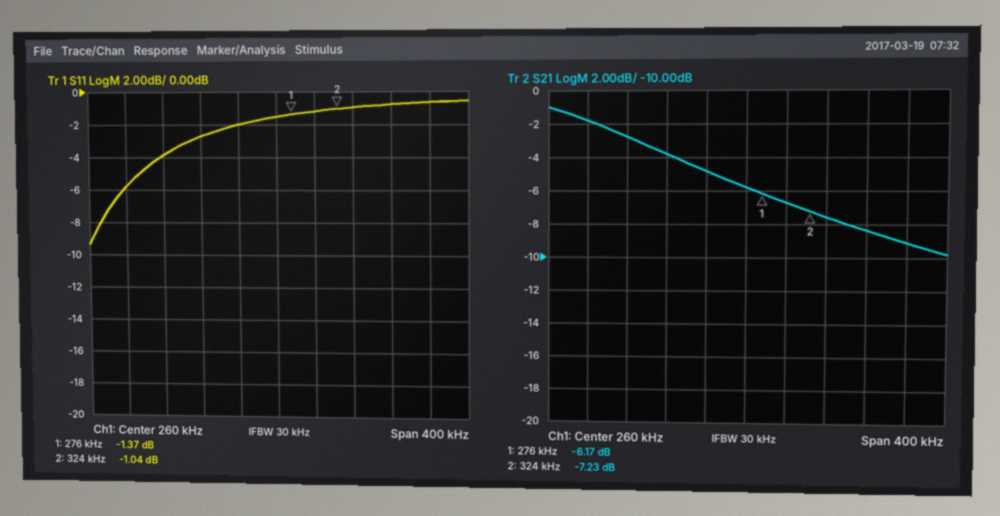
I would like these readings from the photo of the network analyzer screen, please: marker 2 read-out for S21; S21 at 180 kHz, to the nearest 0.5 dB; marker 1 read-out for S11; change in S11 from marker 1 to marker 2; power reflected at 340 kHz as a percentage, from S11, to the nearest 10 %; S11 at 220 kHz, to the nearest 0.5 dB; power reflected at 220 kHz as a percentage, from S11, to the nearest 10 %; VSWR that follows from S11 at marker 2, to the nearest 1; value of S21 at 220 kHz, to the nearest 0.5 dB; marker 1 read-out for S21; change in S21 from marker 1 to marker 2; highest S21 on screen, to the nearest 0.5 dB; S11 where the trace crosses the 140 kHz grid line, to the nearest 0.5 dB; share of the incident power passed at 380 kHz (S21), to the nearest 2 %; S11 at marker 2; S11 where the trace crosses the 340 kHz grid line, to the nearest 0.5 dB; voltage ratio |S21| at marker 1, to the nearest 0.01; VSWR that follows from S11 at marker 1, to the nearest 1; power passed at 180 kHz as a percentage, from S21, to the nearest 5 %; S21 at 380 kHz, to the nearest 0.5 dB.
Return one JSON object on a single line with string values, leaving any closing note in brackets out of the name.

{"marker 2 read-out for S21": "-7.23 dB", "S21 at 180 kHz, to the nearest 0.5 dB": "-4.0 dB", "marker 1 read-out for S11": "-1.37 dB", "change in S11 from marker 1 to marker 2": "0.33 dB", "power reflected at 340 kHz as a percentage, from S11, to the nearest 10 %": "80 %", "S11 at 220 kHz, to the nearest 0.5 dB": "-2.0 dB", "power reflected at 220 kHz as a percentage, from S11, to the nearest 10 %": "60 %", "VSWR that follows from S11 at marker 2, to the nearest 1": "17", "value of S21 at 220 kHz, to the nearest 0.5 dB": "-5.0 dB", "marker 1 read-out for S21": "-6.17 dB", "change in S21 from marker 1 to marker 2": "-1.06 dB", "highest S21 on screen, to the nearest 0.5 dB": "-1.0 dB", "S11 where the trace crosses the 140 kHz grid line, to the nearest 0.5 dB": "-4.0 dB", "share of the incident power passed at 380 kHz (S21), to the nearest 2 %": "14 %", "S11 at marker 2": "-1.04 dB", "S11 where the trace crosses the 340 kHz grid line, to the nearest 0.5 dB": "-1.0 dB", "voltage ratio |S21| at marker 1, to the nearest 0.01": "0.49", "VSWR that follows from S11 at marker 1, to the nearest 1": "13", "power passed at 180 kHz as a percentage, from S21, to the nearest 5 %": "40 %", "S21 at 380 kHz, to the nearest 0.5 dB": "-8.5 dB"}
